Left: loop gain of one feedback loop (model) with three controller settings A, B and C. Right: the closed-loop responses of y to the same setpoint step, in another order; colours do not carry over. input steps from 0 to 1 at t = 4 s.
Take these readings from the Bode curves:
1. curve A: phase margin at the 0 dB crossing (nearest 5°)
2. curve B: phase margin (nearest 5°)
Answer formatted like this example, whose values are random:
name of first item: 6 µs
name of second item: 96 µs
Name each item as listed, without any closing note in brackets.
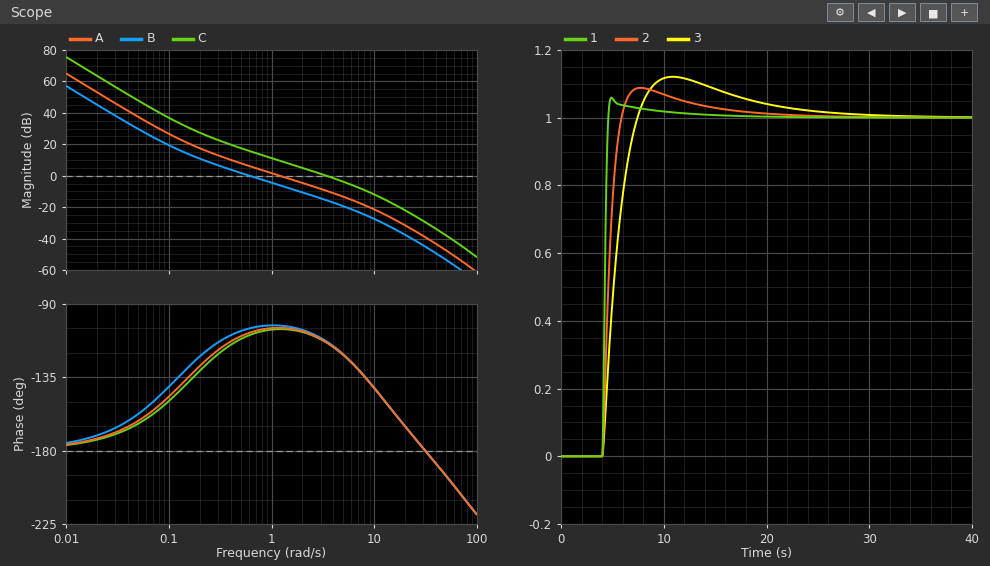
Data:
curve A: phase margin at the 0 dB crossing: 75°
curve B: phase margin: 75°
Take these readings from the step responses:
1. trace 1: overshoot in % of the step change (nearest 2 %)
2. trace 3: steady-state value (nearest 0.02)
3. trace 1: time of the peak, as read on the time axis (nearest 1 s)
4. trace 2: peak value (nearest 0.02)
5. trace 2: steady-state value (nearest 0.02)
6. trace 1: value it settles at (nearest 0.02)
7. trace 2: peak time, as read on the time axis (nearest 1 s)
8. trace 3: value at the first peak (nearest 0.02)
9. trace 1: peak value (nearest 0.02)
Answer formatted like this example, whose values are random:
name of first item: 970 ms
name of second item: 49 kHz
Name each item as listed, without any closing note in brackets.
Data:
trace 1: overshoot in % of the step change: 6 %
trace 3: steady-state value: 1.00
trace 1: time of the peak, as read on the time axis: 5 s
trace 2: peak value: 1.08
trace 2: steady-state value: 1.00
trace 1: value it settles at: 1.00
trace 2: peak time, as read on the time axis: 8 s
trace 3: value at the first peak: 1.12
trace 1: peak value: 1.06
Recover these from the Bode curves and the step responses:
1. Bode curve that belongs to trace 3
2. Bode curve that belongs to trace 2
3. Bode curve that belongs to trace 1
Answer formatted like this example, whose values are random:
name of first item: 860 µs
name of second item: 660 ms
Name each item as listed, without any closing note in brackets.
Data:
Bode curve that belongs to trace 3: B
Bode curve that belongs to trace 2: A
Bode curve that belongs to trace 1: C
